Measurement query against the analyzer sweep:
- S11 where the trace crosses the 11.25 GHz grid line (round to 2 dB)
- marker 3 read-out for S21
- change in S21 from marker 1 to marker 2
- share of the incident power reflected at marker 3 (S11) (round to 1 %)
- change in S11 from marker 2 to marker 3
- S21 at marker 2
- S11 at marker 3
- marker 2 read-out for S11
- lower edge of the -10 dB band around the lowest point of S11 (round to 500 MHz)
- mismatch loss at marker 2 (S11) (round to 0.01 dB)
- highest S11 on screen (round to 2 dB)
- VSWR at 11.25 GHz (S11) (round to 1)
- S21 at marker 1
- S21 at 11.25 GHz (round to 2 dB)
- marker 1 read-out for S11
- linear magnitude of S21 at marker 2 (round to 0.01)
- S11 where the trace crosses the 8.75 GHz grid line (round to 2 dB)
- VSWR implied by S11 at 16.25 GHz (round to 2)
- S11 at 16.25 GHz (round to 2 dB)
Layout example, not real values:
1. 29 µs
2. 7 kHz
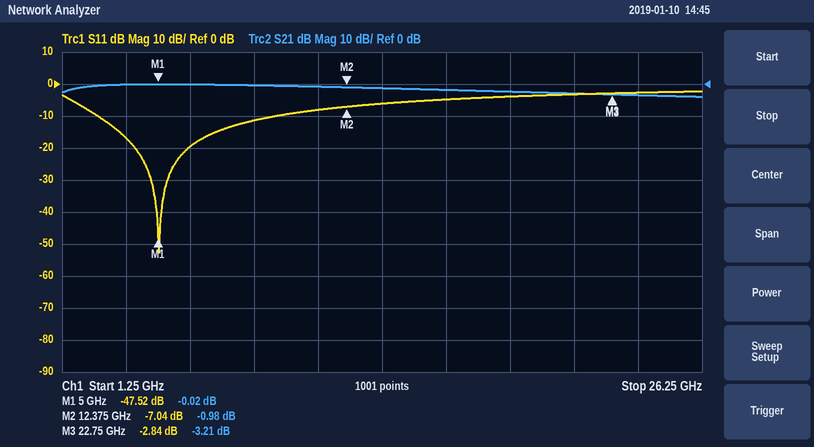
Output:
1. -8 dB
2. -3.21 dB
3. -0.96 dB
4. 52 %
5. 4.20 dB
6. -0.98 dB
7. -2.84 dB
8. -7.04 dB
9. 2.5 GHz
10. 0.96 dB
11. -2 dB
12. 2
13. -0.02 dB
14. 0 dB
15. -47.52 dB
16. 0.89
17. -12 dB
18. 4
19. -4 dB
